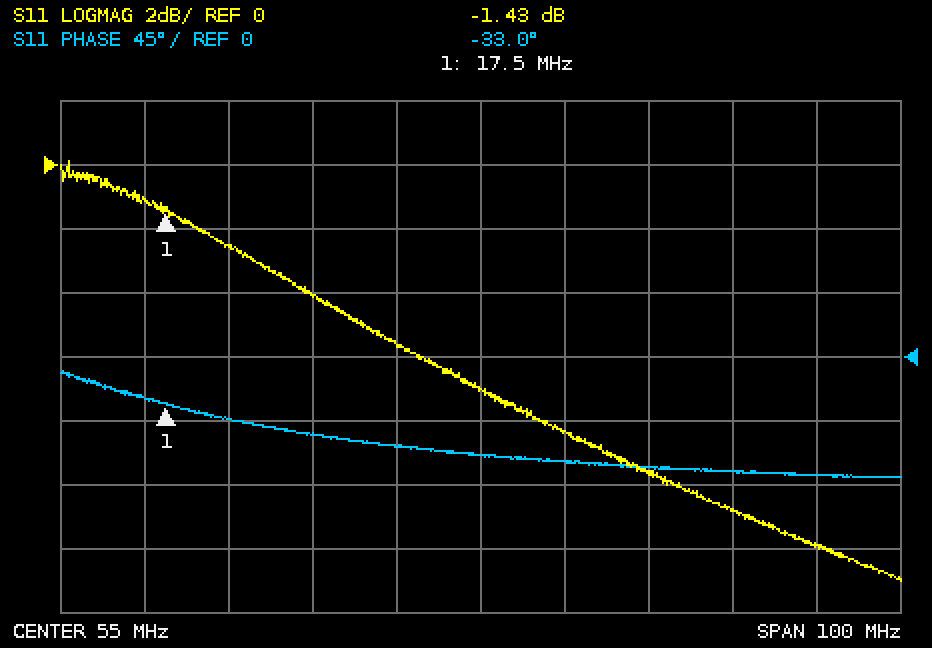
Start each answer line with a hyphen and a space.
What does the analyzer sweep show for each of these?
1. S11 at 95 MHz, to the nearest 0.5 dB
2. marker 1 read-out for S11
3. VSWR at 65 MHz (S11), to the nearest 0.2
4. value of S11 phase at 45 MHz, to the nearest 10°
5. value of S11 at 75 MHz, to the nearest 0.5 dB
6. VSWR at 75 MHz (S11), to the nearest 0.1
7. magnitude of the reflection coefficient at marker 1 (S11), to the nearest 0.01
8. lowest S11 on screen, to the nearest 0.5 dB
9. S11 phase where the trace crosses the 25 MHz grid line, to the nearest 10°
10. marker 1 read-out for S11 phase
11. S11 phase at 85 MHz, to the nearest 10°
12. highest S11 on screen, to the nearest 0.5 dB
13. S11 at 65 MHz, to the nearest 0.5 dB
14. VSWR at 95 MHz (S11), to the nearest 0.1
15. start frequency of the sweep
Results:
- -12.0 dB
- -1.43 dB
- 2.2
- -60°
- -9.5 dB
- 2.0
- 0.85
- -13.0 dB
- -40°
- -33.0°
- -80°
- 0.0 dB
- -8.5 dB
- 1.7
- 5 MHz
